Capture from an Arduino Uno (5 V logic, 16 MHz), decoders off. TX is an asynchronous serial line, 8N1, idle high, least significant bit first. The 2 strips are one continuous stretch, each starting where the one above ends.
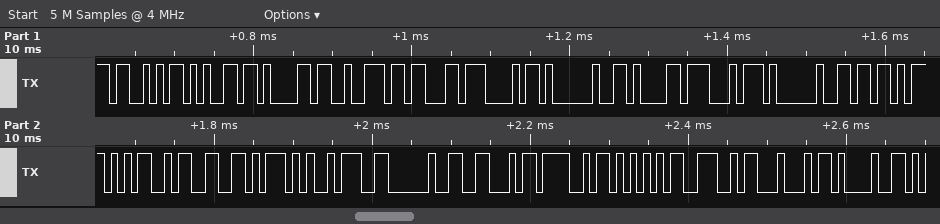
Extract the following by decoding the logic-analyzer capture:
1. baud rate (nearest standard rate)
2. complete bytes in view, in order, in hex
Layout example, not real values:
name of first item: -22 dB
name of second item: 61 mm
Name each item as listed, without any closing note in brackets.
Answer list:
baud rate: 115200 baud
complete bytes in view, in order, in hex: 53 65 61 72 63 68 20 61 74 20 5B 35 33 5D 3A 20 46 4F 55 4E 44 21
